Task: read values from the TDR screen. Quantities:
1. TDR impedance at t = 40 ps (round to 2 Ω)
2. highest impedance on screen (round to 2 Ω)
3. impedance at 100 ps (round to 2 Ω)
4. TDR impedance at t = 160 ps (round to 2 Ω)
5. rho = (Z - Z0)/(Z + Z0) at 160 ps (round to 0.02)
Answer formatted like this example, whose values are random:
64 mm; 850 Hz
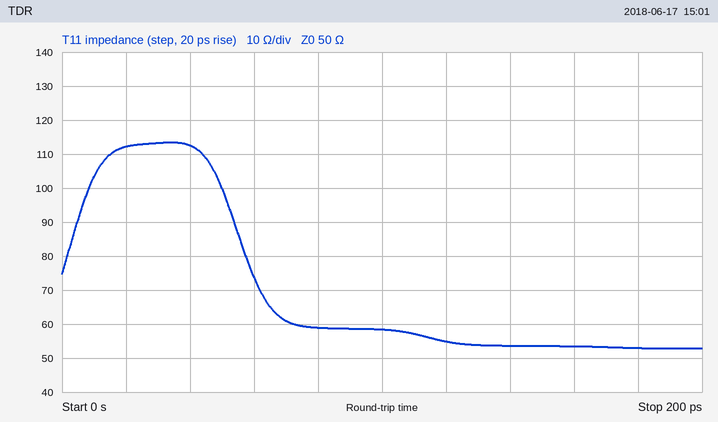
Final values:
112 Ω; 114 Ω; 58 Ω; 54 Ω; +0.04
